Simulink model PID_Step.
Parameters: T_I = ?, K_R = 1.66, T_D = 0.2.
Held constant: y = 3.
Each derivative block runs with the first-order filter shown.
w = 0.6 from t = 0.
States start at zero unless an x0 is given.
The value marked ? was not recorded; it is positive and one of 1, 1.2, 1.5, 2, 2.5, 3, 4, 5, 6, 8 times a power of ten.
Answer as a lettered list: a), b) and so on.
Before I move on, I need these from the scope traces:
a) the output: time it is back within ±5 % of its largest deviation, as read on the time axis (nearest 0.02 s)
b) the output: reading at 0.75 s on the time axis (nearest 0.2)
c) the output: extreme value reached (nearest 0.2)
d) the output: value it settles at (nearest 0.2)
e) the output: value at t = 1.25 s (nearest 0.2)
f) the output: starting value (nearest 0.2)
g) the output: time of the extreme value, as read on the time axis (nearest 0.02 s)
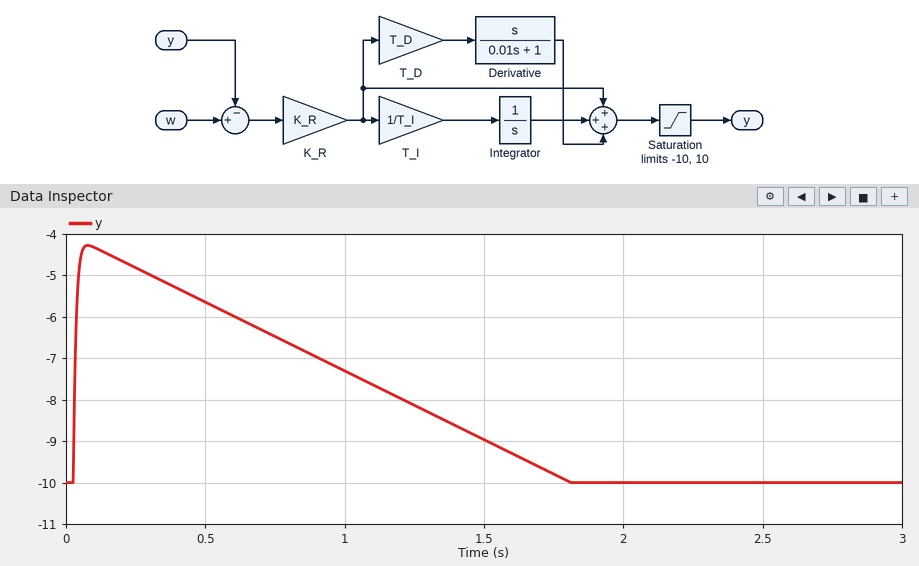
a) 1.72 s
b) -6.4
c) -4.2
d) -10.0
e) -8.2
f) -10.0
g) 0.08 s
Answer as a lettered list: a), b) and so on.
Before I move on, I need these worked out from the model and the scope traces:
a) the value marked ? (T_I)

a) 1.2
